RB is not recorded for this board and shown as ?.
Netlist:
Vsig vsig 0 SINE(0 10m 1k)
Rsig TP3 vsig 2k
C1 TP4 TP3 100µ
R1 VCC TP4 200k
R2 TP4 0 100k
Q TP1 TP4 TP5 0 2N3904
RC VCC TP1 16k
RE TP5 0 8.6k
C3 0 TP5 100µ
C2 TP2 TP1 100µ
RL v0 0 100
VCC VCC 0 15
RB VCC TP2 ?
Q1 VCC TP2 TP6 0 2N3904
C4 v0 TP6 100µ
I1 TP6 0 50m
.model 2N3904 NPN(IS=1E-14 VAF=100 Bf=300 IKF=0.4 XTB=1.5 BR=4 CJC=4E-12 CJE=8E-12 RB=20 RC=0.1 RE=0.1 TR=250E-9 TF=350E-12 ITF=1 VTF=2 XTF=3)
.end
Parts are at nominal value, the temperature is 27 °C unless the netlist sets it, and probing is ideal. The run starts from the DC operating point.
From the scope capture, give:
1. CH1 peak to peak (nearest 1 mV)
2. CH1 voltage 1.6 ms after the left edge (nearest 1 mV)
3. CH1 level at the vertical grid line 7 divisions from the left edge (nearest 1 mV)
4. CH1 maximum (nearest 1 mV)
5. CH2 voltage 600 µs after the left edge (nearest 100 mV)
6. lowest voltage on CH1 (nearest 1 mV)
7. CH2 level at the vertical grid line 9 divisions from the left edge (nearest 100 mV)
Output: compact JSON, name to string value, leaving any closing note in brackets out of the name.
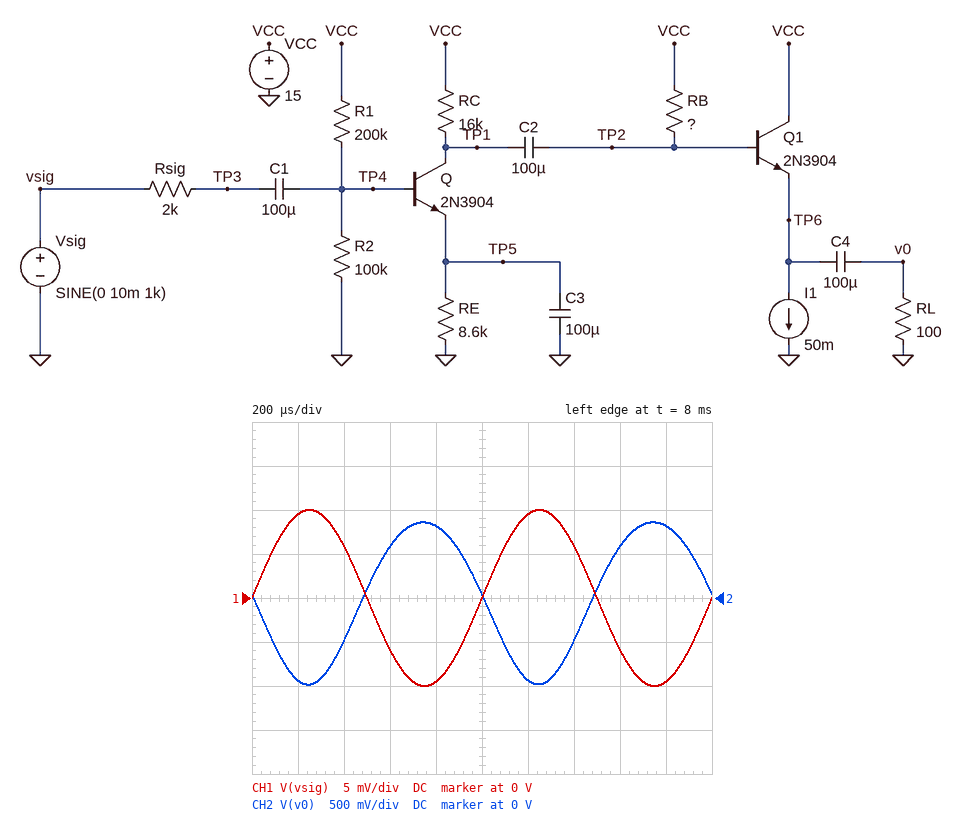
{"CH1 peak to peak": "20 mV", "CH1 voltage 1.6 ms after the left edge": "-6 mV", "CH1 level at the vertical grid line 7 divisions from the left edge": "6 mV", "CH1 maximum": "10 mV", "CH2 voltage 600 µs after the left edge": "600 mV", "lowest voltage on CH1": "-10 mV", "CH2 level at the vertical grid line 9 divisions from the left edge": "800 mV"}
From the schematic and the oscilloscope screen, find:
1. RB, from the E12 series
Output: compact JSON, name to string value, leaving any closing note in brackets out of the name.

{"RB, from the E12 series": "15 kΩ"}
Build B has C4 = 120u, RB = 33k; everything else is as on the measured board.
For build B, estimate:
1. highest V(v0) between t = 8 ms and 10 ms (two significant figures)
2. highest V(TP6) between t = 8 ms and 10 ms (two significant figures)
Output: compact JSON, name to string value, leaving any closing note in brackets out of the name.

{"highest V(v0) between t = 8 ms and 10 ms": "1.1 V", "highest V(TP6) between t = 8 ms and 10 ms": "9.5 V"}
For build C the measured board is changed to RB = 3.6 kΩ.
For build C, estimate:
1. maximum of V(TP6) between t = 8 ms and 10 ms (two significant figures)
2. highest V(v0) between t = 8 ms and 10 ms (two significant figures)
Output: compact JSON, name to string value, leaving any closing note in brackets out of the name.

{"maximum of V(TP6) between t = 8 ms and 10 ms": "14 V", "highest V(v0) between t = 8 ms and 10 ms": "390 mV"}
